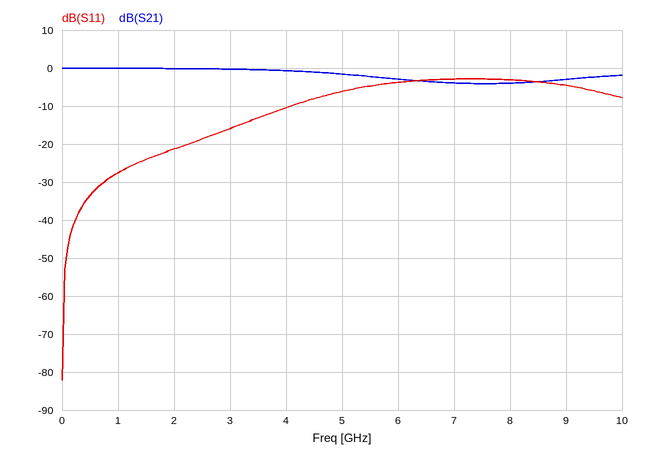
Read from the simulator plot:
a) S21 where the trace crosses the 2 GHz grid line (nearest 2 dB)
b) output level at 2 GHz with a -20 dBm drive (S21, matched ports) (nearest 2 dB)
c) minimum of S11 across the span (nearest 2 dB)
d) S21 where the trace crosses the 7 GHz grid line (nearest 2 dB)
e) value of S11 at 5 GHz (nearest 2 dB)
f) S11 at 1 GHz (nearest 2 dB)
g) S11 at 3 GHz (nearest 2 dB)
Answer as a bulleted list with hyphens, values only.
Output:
- 0 dB
- -20 dBm
- -82 dB
- -4 dB
- -6 dB
- -28 dB
- -16 dB
